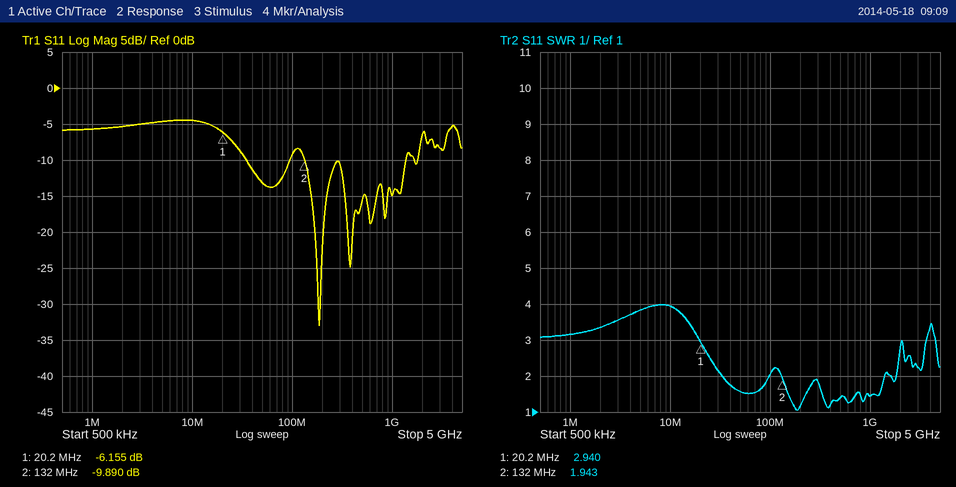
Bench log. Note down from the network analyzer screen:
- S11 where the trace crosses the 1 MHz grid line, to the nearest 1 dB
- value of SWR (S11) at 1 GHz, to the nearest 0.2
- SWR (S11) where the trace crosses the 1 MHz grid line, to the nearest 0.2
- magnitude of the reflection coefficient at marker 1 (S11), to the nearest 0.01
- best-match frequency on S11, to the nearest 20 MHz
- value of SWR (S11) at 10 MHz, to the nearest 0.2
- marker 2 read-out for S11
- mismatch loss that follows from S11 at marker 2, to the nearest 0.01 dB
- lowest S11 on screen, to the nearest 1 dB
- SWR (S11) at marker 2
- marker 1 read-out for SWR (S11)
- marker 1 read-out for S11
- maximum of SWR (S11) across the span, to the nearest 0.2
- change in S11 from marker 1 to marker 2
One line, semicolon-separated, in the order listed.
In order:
-6 dB; 1.4; 3.2; 0.49; 180 MHz; 4.0; -9.890 dB; 0.47 dB; -33 dB; 1.943; 2.940; -6.155 dB; 4.0; -3.735 dB
